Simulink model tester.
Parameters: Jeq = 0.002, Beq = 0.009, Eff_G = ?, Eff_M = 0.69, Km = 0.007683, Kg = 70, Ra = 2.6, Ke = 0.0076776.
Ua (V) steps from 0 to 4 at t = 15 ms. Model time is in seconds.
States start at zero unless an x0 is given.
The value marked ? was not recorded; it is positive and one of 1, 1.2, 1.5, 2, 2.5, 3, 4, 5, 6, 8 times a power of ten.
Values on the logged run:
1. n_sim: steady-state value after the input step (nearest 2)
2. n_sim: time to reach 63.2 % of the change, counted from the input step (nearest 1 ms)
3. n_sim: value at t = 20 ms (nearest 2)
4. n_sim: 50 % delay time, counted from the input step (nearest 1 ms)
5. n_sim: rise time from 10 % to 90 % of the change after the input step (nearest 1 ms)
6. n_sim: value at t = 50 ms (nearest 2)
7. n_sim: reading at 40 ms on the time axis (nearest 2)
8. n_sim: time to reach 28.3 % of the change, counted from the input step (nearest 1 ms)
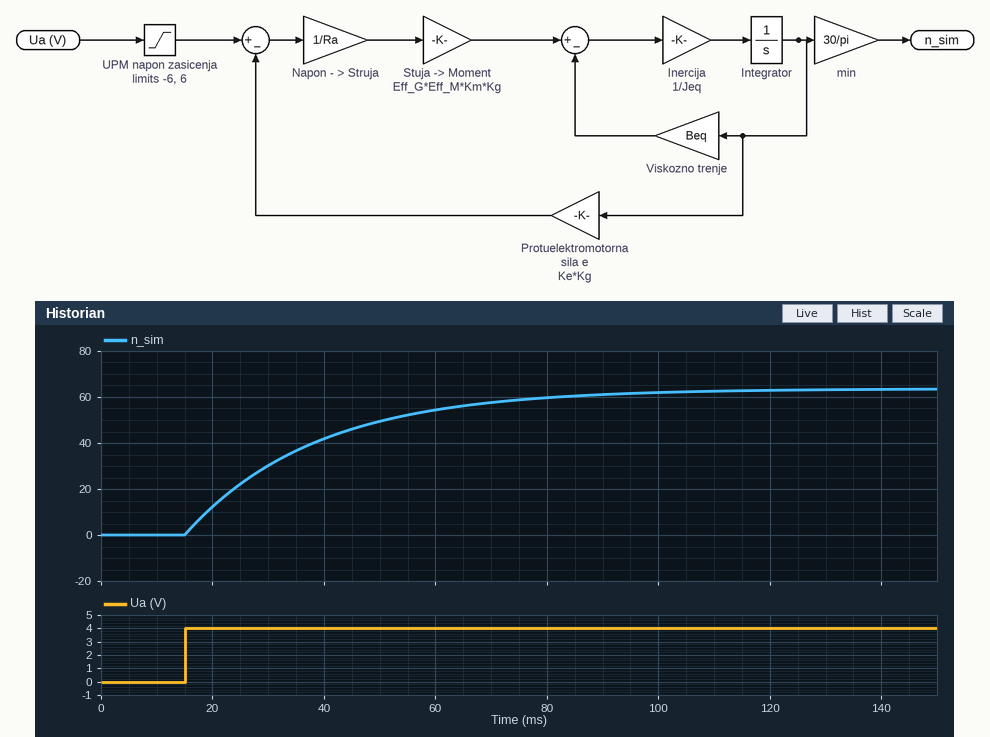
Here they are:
64
23 ms
12
16 ms
51 ms
50
42
8 ms
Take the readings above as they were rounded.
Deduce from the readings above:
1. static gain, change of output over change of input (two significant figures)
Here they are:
16
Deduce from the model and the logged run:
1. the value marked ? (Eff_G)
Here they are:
1
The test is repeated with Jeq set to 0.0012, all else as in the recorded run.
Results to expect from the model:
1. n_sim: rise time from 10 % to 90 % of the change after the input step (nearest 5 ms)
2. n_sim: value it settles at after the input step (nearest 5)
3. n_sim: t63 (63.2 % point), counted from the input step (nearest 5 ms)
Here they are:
30 ms
65
15 ms
